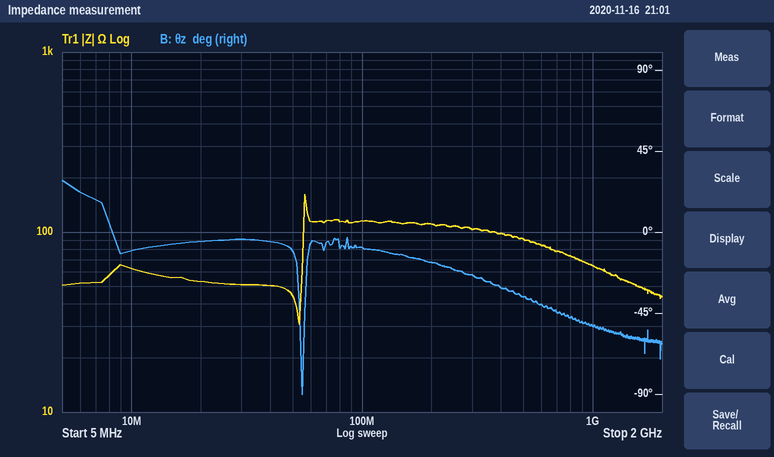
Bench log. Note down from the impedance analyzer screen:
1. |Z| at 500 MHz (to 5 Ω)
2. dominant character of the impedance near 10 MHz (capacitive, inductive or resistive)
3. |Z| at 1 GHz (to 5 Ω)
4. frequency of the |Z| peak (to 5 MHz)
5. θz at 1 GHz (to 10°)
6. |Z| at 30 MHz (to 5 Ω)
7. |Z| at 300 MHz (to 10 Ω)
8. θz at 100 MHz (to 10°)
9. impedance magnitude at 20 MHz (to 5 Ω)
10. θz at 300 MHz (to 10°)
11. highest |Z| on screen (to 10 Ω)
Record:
90 Ω
resistive
65 Ω
55 MHz
-50°
50 Ω
100 Ω
-10°
55 Ω
-20°
160 Ω
